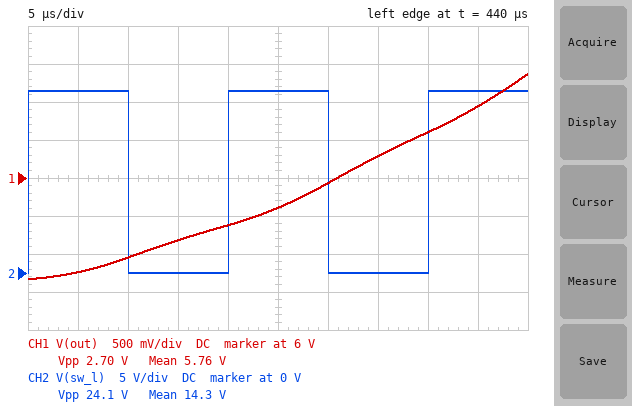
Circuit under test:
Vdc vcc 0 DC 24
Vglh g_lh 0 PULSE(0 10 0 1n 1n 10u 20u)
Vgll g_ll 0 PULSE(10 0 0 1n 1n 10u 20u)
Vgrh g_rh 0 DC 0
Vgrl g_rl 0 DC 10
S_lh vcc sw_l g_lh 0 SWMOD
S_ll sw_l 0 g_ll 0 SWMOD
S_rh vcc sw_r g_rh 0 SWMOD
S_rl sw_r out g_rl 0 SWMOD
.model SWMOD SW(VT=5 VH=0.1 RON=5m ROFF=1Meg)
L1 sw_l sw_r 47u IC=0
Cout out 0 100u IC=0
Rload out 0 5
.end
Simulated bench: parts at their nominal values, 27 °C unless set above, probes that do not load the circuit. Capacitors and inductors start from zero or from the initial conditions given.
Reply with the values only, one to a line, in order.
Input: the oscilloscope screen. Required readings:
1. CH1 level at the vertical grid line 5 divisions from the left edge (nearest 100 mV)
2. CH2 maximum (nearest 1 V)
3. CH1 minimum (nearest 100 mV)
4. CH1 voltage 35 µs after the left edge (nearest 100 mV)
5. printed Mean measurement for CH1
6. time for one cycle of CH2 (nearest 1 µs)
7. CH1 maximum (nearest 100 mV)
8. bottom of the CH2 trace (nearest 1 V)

5.6 V
24 V
4.7 V
6.3 V
5.76 V
20 µs
7.4 V
0 V
